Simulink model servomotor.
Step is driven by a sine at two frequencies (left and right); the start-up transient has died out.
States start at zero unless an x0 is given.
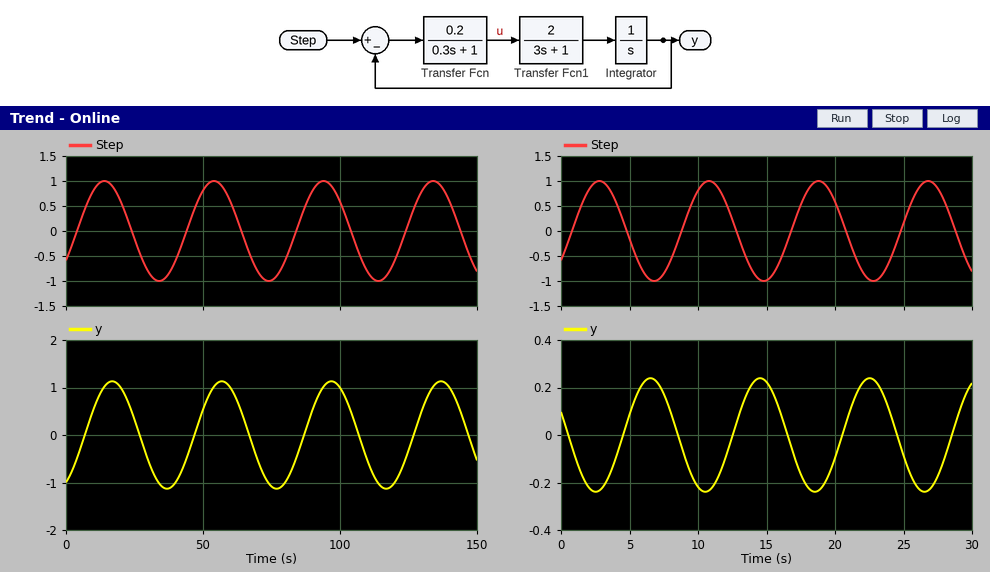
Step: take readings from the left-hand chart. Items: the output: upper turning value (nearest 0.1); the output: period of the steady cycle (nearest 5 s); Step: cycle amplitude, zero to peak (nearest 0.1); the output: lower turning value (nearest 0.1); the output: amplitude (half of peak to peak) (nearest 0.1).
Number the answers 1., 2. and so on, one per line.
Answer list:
1. 1.1
2. 40 s
3. 1.0
4. -1.1
5. 1.1
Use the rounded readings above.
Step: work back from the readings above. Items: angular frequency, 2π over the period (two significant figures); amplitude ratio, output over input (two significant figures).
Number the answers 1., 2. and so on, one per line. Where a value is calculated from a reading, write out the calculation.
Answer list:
1. 2π / 40 = 0.16 rad/s
2. 1.1 / 1 = 1.1
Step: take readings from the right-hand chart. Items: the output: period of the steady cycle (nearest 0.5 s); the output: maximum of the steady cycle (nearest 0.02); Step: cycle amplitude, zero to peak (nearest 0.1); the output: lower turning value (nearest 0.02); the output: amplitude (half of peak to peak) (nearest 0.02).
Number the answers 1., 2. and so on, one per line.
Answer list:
1. 8.0 s
2. 0.24
3. 1.0
4. -0.24
5. 0.24
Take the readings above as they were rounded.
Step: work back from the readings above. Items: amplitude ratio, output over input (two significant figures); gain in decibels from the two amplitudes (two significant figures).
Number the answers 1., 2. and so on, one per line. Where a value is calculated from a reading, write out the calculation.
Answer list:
1. 0.24 / 1 = 0.24
2. 20 log10(0.24 / 1) = -12 dB
